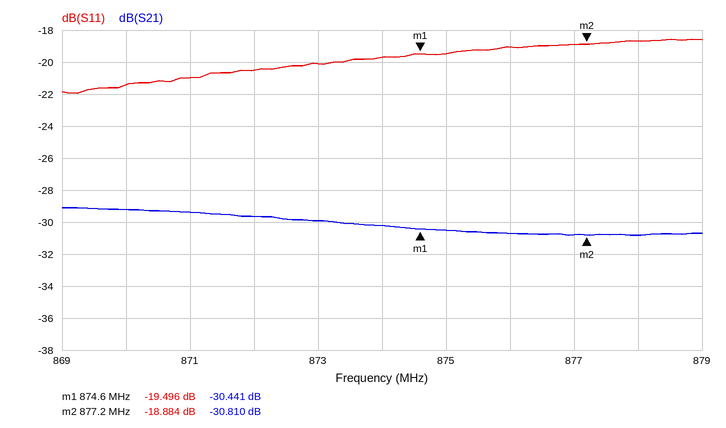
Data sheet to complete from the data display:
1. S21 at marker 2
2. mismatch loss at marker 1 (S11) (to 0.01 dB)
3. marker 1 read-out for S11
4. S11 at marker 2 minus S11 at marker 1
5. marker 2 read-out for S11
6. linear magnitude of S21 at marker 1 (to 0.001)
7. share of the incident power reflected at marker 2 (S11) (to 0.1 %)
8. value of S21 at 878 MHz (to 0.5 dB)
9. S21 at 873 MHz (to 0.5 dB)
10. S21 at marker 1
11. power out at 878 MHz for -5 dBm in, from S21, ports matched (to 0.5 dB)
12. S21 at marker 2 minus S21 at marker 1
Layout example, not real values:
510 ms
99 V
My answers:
-30.810 dB
0.05 dB
-19.496 dB
0.612 dB
-18.884 dB
0.030
1.3 %
-31.0 dB
-30.0 dB
-30.441 dB
-36.0 dBm
-0.369 dB
